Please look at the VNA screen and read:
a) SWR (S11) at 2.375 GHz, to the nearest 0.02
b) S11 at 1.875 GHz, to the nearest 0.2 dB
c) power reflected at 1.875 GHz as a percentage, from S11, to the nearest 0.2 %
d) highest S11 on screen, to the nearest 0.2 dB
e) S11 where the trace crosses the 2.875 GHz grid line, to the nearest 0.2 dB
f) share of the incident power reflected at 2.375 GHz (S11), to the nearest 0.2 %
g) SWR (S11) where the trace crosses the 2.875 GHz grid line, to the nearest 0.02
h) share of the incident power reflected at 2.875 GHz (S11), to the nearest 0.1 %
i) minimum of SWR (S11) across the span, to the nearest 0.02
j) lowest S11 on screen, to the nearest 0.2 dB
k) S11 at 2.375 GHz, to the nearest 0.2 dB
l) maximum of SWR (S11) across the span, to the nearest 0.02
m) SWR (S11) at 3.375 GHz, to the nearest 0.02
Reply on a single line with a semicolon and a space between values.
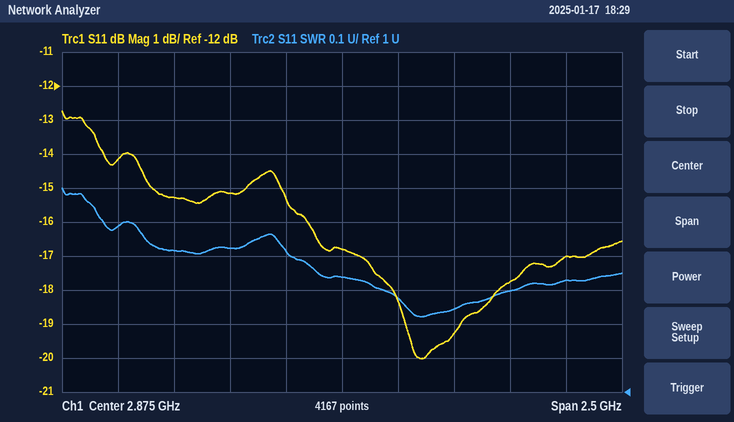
1.42; -14.2 dB; 3.8 %; -12.8 dB; -16.8 dB; 3.0 %; 1.34; 2.1 %; 1.22; -20.0 dB; -15.2 dB; 1.60; 1.24
